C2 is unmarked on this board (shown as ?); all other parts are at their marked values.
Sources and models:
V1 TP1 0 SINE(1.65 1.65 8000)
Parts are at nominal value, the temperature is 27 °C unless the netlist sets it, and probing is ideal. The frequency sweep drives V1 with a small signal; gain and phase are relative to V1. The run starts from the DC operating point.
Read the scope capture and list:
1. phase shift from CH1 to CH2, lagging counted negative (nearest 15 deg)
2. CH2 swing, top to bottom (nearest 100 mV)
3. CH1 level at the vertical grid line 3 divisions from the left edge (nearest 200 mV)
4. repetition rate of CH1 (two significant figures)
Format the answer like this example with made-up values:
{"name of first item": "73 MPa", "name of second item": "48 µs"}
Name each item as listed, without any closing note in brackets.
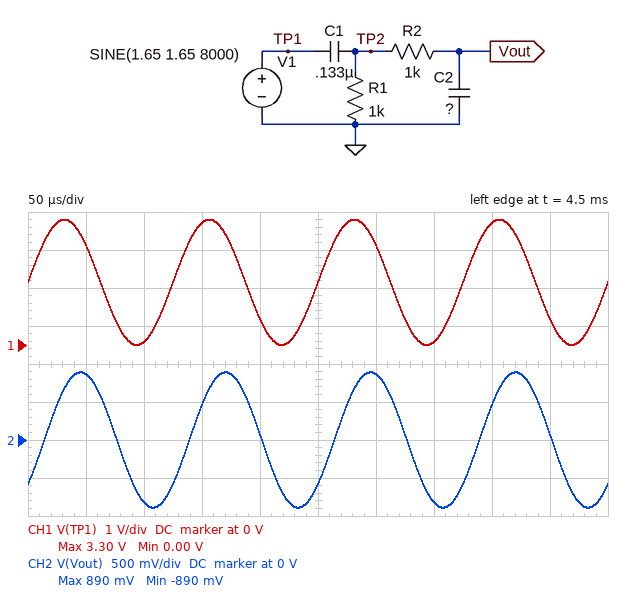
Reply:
{"phase shift from CH1 to CH2, lagging counted negative": "-45 deg", "CH2 swing, top to bottom": "1.8 V", "CH1 level at the vertical grid line 3 divisions from the left edge": "3.2 V", "repetition rate of CH1": "8.0 kHz"}
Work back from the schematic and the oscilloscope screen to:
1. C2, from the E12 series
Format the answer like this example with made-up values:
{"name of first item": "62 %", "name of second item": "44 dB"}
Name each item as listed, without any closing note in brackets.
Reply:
{"C2, from the E12 series": "27 nF"}
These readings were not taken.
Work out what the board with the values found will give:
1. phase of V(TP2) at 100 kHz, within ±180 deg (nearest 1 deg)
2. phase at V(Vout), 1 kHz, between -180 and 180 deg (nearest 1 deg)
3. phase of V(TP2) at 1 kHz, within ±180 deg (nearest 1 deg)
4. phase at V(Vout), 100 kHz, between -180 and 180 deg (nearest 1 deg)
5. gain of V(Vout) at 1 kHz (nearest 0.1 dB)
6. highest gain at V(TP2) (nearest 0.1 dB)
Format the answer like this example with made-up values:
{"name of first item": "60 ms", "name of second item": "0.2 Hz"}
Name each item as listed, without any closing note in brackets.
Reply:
{"phase of V(TP2) at 100 kHz, within ±180 deg": "1 deg", "phase at V(Vout), 1 kHz, between -180 and 180 deg": "36 deg", "phase of V(TP2) at 1 kHz, within ±180 deg": "46 deg", "phase at V(Vout), 100 kHz, between -180 and 180 deg": "-85 deg", "gain of V(Vout) at 1 kHz": "-4.8 dB", "highest gain at V(TP2)": "0 dB"}
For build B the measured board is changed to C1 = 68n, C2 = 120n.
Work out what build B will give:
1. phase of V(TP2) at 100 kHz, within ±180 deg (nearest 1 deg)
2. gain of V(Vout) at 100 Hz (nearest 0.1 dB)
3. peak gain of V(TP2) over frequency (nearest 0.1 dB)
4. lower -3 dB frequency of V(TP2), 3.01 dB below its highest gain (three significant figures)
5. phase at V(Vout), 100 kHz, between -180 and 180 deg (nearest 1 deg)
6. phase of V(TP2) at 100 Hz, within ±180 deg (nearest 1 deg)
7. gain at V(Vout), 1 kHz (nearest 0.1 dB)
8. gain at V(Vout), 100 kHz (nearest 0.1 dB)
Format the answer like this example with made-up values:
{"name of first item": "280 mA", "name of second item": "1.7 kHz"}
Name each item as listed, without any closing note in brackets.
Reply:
{"phase of V(TP2) at 100 kHz, within ±180 deg": "3 deg", "gain of V(Vout) at 100 Hz": "-27.5 dB", "peak gain of V(TP2) over frequency": "0 dB", "lower -3 dB frequency of V(TP2), 3.01 dB below its highest gain": "5.17 kHz", "phase at V(Vout), 100 kHz, between -180 and 180 deg": "-87 deg", "phase of V(TP2) at 100 Hz, within ±180 deg": "83 deg", "gain at V(Vout), 1 kHz": "-13.6 dB", "gain at V(Vout), 100 kHz": "-37.6 dB"}
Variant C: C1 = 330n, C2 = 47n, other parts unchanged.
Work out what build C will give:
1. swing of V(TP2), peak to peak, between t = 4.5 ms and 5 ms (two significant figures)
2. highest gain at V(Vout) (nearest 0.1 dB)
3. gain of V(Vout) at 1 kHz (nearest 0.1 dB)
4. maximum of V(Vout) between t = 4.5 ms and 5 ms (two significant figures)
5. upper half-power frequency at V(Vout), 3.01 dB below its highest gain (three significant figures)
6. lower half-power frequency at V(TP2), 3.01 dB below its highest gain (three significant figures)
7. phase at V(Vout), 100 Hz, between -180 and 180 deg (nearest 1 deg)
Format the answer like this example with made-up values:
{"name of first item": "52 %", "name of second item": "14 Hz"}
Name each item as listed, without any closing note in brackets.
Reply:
{"swing of V(TP2), peak to peak, between t = 4.5 ms and 5 ms": "3.2 V", "highest gain at V(Vout)": "-2.2 dB", "gain of V(Vout) at 1 kHz": "-2.3 dB", "maximum of V(Vout) between t = 4.5 ms and 5 ms": "630 mV", "upper half-power frequency at V(Vout), 3.01 dB below its highest gain": "4.70 kHz", "lower half-power frequency at V(TP2), 3.01 dB below its highest gain": "592 Hz", "phase at V(Vout), 100 Hz, between -180 and 180 deg": "75 deg"}
